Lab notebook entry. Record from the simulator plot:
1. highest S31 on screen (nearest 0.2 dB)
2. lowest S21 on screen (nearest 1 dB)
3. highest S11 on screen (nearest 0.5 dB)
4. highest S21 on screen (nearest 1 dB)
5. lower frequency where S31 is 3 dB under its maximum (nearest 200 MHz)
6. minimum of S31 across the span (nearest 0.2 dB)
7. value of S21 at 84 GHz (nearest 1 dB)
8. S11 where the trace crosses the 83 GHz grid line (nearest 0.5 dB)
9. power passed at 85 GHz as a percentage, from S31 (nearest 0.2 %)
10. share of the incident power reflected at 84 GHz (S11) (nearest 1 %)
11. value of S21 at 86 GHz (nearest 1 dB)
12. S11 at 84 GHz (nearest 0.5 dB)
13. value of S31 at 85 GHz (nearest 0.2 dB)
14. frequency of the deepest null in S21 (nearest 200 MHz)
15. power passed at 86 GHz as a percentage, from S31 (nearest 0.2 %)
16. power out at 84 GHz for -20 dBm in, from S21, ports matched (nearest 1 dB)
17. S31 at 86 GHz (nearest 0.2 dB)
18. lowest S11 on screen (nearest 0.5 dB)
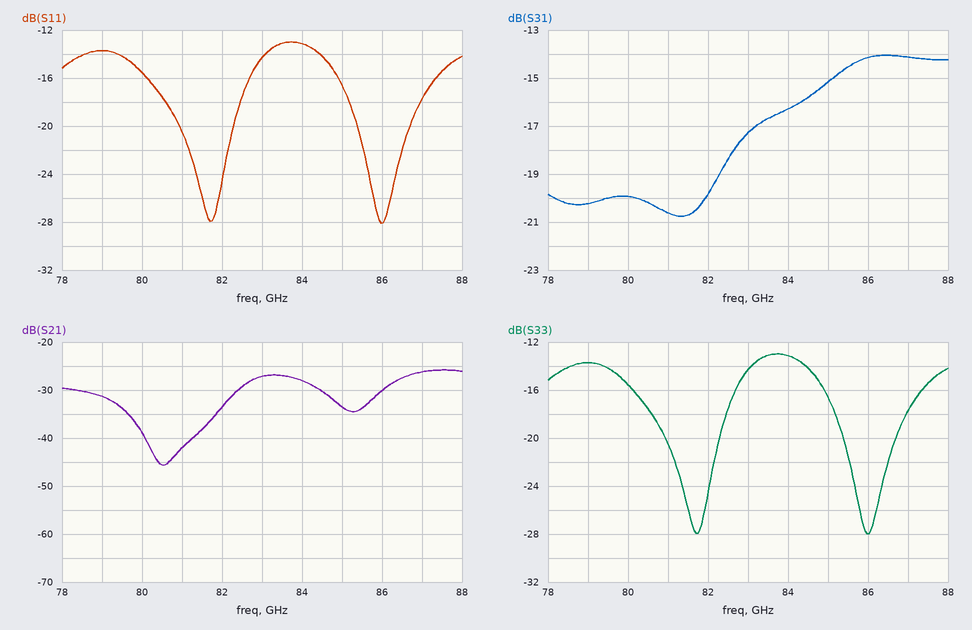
-14.0 dB
-46 dB
-13.0 dB
-26 dB
83.2 GHz
-20.8 dB
-28 dB
-14.5 dB
3.0 %
5 %
-30 dB
-13.0 dB
-15.2 dB
80.6 GHz
3.8 %
-48 dBm
-14.2 dB
-28.0 dB
